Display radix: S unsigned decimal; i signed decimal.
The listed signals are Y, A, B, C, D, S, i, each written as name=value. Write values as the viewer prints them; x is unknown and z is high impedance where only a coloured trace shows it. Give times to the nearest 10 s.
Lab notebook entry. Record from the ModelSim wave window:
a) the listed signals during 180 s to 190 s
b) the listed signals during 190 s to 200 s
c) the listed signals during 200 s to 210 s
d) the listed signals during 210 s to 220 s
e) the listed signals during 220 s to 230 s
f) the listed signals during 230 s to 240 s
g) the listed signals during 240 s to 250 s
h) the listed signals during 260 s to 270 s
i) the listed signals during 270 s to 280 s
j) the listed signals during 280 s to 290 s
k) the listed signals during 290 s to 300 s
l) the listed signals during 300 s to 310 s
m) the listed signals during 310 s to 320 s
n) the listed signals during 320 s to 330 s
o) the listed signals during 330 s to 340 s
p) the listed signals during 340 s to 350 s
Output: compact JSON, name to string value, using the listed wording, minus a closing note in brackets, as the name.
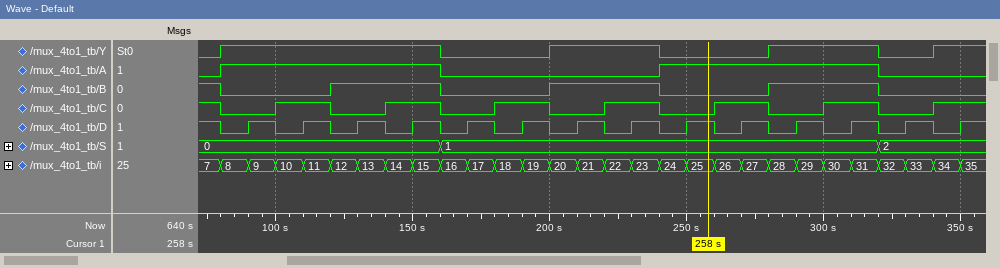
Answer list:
{"the listed signals during 180 s to 190 s": "Y=0, A=0, B=0, C=1, D=0, S=1, i=18", "the listed signals during 190 s to 200 s": "Y=0, A=0, B=0, C=1, D=1, S=1, i=19", "the listed signals during 200 s to 210 s": "Y=1, A=0, B=1, C=0, D=0, S=1, i=20", "the listed signals during 210 s to 220 s": "Y=1, A=0, B=1, C=0, D=1, S=1, i=21", "the listed signals during 220 s to 230 s": "Y=1, A=0, B=1, C=1, D=0, S=1, i=22", "the listed signals during 230 s to 240 s": "Y=1, A=0, B=1, C=1, D=1, S=1, i=23", "the listed signals during 240 s to 250 s": "Y=0, A=1, B=0, C=0, D=0, S=1, i=24", "the listed signals during 260 s to 270 s": "Y=0, A=1, B=0, C=1, D=0, S=1, i=26", "the listed signals during 270 s to 280 s": "Y=0, A=1, B=0, C=1, D=1, S=1, i=27", "the listed signals during 280 s to 290 s": "Y=1, A=1, B=1, C=0, D=0, S=1, i=28", "the listed signals during 290 s to 300 s": "Y=1, A=1, B=1, C=0, D=1, S=1, i=29", "the listed signals during 300 s to 310 s": "Y=1, A=1, B=1, C=1, D=0, S=1, i=30", "the listed signals during 310 s to 320 s": "Y=1, A=1, B=1, C=1, D=1, S=1, i=31", "the listed signals during 320 s to 330 s": "Y=0, A=0, B=0, C=0, D=0, S=2, i=32", "the listed signals during 330 s to 340 s": "Y=0, A=0, B=0, C=0, D=1, S=2, i=33", "the listed signals during 340 s to 350 s": "Y=1, A=0, B=0, C=1, D=0, S=2, i=34"}
